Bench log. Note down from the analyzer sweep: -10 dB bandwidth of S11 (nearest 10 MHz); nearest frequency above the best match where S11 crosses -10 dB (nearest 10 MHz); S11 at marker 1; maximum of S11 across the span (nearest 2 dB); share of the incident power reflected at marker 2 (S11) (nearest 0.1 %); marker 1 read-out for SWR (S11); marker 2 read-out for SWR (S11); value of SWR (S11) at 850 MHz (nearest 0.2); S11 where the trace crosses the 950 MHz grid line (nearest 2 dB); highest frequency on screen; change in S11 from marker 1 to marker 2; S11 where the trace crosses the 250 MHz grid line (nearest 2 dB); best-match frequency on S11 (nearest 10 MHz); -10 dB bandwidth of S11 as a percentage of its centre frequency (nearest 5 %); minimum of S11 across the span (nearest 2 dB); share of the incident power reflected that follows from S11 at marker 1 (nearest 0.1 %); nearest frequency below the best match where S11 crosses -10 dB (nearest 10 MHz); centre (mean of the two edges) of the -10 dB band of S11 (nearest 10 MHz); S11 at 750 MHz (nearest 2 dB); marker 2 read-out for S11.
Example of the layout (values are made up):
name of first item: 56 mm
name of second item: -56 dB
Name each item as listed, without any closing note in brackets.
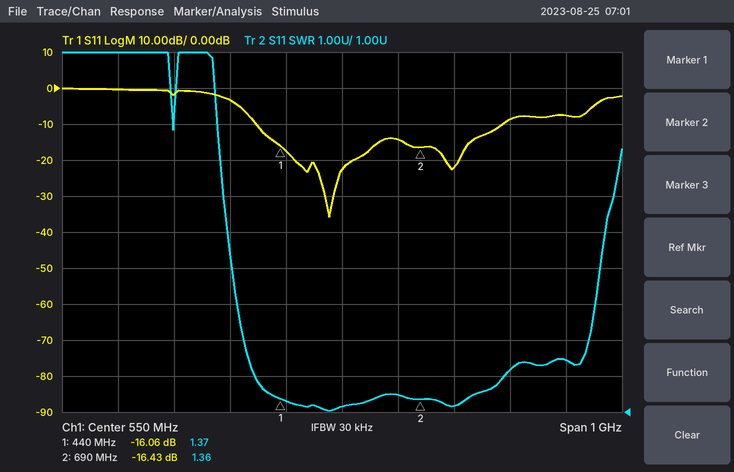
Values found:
-10 dB bandwidth of S11: 440 MHz
nearest frequency above the best match where S11 crosses -10 dB: 840 MHz
S11 at marker 1: -16.06 dB
maximum of S11 across the span: 0 dB
share of the incident power reflected at marker 2 (S11): 2.3 %
marker 1 read-out for SWR: 1.37
marker 2 read-out for SWR: 1.36
value of SWR (S11) at 850 MHz: 2.2
S11 where the trace crosses the 950 MHz grid line: -8 dB
highest frequency on screen: 1.05 GHz
change in S11 from marker 1 to marker 2: -0.37 dB
S11 where the trace crosses the 250 MHz grid line: -2 dB
best-match frequency on S11: 530 MHz
-10 dB bandwidth of S11 as a percentage of its centre frequency: 70 %
minimum of S11 across the span: -36 dB
share of the incident power reflected that follows from S11 at marker 1: 2.5 %
nearest frequency below the best match where S11 crosses -10 dB: 400 MHz
centre (mean of the two edges) of the -10 dB band of S11: 620 MHz
S11 at 750 MHz: -22 dB
marker 2 read-out for S11: -16.43 dB
